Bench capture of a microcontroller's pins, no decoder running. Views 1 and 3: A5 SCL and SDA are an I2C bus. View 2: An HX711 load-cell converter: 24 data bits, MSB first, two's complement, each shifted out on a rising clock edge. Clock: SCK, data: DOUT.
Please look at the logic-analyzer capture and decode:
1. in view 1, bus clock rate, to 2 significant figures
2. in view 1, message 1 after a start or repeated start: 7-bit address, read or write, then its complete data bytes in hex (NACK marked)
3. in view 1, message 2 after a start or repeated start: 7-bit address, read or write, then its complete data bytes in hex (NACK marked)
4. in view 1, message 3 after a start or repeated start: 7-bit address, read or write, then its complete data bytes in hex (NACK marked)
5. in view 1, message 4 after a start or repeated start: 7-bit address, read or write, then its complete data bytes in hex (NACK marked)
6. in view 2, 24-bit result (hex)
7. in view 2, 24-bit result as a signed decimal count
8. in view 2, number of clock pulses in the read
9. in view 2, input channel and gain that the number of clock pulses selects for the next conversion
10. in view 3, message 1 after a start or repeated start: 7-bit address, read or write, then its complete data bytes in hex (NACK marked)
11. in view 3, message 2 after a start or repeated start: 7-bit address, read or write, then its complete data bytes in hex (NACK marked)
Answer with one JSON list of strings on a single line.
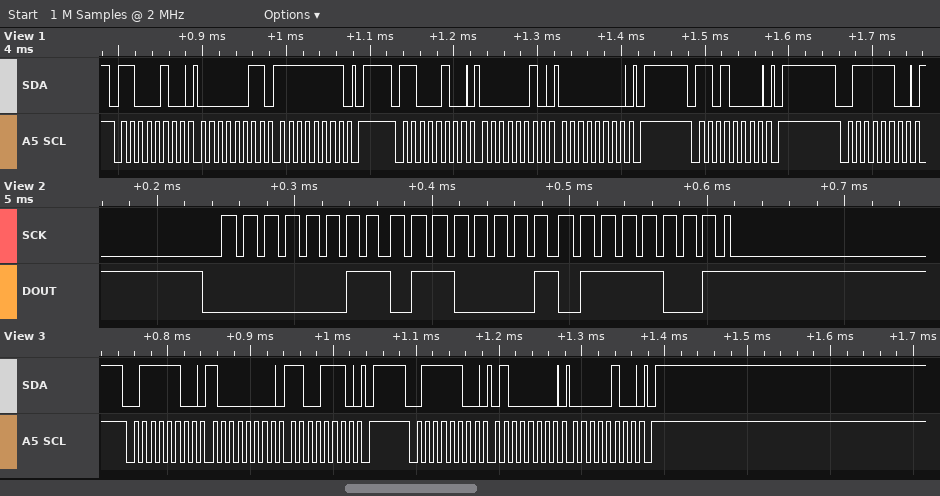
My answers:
["100 kHz", "0x62 write: 03 FF", "0x62 write: 02 00", "0x68 write", "0x3E write", "0x036179", "221561", "25", "channel A, gain 128", "0x3E write: 80 CE", "0x3E write: 40 04"]
